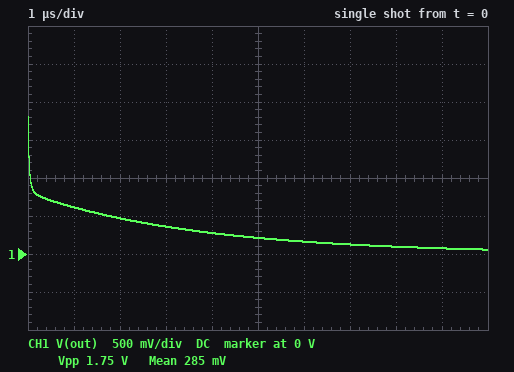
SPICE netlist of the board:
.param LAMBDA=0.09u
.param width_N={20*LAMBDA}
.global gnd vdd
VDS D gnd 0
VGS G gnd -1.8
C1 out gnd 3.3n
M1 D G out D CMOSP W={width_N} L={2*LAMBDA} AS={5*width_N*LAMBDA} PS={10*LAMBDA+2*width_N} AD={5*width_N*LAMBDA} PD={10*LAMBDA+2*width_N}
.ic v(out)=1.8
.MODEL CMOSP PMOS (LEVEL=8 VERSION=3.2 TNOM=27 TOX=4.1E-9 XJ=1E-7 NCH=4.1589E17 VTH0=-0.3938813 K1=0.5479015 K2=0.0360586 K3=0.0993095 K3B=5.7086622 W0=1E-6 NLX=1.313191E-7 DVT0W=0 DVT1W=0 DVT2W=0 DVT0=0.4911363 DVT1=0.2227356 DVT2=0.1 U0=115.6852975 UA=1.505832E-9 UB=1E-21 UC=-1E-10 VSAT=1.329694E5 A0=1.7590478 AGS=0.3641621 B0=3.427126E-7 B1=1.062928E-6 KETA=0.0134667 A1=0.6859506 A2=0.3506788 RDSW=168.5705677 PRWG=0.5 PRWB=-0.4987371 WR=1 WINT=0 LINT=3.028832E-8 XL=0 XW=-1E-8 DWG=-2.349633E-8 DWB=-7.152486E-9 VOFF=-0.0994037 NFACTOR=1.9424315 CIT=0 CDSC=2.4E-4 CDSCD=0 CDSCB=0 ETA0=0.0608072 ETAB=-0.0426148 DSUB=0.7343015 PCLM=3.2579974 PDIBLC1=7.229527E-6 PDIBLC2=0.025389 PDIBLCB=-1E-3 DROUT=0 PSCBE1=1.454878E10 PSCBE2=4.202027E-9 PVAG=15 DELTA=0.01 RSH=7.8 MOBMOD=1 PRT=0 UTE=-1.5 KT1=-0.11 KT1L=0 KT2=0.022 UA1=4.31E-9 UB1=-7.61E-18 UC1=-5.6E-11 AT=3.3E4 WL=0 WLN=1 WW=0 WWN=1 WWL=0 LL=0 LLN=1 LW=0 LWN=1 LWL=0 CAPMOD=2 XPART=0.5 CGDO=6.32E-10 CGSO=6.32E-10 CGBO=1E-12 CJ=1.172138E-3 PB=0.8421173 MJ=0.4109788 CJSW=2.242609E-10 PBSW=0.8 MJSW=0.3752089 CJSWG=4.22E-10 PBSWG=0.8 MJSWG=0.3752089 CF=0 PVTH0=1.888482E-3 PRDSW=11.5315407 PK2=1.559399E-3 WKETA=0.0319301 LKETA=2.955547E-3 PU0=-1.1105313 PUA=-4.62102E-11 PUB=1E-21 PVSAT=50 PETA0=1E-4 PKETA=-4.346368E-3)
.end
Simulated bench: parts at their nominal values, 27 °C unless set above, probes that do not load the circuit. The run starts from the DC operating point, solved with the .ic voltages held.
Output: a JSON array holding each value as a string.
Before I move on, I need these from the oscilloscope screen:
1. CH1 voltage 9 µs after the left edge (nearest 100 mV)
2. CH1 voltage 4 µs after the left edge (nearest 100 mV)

["100 mV", "300 mV"]
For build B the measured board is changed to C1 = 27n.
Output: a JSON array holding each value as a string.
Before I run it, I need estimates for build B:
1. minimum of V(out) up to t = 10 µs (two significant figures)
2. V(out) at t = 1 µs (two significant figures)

["580 mV", "830 mV"]
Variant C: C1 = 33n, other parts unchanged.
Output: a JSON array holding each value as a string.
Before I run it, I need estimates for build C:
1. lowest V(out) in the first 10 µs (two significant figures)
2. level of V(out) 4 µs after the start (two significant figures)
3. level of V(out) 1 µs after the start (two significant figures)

["610 mV", "720 mV", "850 mV"]
